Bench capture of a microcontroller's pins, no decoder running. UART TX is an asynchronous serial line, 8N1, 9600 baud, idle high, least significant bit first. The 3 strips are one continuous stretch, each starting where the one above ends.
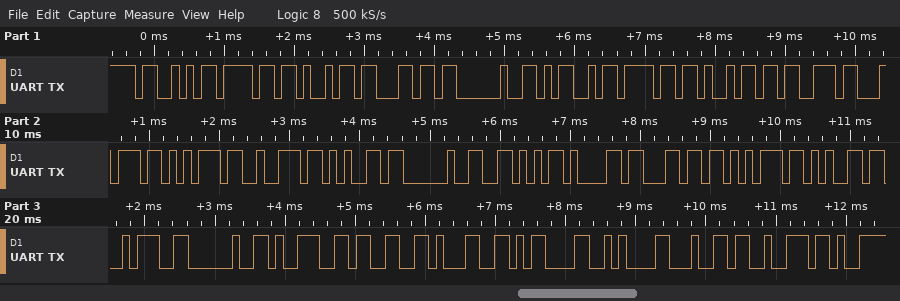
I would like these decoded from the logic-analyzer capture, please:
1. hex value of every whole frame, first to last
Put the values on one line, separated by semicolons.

53 6F 69 6C 20 4D 6F 69 73 74 75 72 65 20 56 61 6C 75 65 3A 20 39 33 31 0D 0A 64 72
